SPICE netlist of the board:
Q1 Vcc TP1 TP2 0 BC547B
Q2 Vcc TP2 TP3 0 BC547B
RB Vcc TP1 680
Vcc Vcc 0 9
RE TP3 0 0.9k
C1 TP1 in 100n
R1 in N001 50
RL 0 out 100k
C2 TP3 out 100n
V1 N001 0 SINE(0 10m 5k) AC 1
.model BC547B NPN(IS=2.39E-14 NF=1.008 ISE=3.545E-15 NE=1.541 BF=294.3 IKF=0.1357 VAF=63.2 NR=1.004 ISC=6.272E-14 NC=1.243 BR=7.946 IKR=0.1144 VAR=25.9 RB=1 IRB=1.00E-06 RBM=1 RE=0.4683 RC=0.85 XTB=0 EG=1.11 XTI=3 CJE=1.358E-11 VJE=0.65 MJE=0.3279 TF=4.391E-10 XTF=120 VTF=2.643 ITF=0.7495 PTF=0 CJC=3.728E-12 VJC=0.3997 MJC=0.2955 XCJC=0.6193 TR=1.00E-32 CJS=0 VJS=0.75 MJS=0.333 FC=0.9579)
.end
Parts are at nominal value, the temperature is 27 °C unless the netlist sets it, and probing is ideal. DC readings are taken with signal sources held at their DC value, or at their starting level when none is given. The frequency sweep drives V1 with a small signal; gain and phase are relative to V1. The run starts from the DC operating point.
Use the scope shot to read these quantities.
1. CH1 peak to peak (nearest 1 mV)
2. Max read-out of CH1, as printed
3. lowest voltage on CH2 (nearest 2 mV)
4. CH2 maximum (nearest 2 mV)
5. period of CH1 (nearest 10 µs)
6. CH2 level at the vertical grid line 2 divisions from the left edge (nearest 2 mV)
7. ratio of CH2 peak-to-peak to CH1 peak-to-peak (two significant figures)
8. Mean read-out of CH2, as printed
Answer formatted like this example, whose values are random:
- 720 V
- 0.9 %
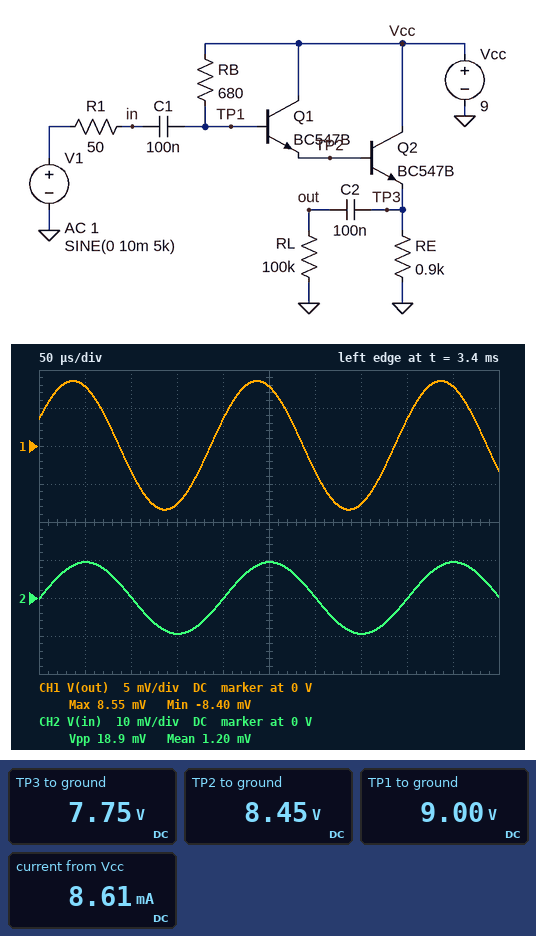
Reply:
- 17 mV
- 8.55 mV
- -10 mV
- 10 mV
- 200 µs
- 0 V
- 1.1
- 1.20 mV
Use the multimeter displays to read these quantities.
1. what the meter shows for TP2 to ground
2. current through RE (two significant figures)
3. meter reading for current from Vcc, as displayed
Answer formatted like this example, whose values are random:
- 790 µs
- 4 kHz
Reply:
- 8.45 V
- 8.6 mA
- 8.61 mA
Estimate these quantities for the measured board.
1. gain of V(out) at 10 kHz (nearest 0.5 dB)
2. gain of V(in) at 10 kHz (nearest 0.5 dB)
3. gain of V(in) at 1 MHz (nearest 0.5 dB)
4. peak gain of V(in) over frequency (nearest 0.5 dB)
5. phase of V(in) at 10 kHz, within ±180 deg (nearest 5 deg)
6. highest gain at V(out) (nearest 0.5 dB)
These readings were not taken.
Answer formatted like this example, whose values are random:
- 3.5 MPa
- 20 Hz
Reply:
- -1.0 dB
- -0.5 dB
- -0.5 dB
- 0 dB
- 0 deg
- -0.5 dB
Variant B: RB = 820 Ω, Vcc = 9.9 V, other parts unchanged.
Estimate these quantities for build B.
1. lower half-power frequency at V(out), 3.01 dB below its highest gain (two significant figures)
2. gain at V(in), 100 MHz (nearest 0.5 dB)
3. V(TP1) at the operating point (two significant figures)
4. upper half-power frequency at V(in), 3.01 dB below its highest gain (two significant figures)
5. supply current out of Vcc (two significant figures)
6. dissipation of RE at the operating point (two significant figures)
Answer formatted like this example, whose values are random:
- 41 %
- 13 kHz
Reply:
- 1.8 kHz
- -0.5 dB
- 9.9 V
- 430 MHz
- 9.6 mA
- 83 mW
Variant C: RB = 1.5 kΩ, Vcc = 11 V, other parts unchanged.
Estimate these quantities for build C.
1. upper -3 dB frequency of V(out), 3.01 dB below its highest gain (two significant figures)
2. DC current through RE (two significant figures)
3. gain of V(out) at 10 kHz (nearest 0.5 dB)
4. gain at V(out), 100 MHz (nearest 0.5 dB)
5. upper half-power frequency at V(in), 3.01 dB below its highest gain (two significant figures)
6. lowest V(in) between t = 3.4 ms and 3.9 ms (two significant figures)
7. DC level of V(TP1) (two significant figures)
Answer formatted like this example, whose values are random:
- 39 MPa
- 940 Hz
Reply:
- 370 MHz
- 11 mA
- -0.5 dB
- -1.5 dB
- 450 MHz
- -9.7 mV
- 11 V
